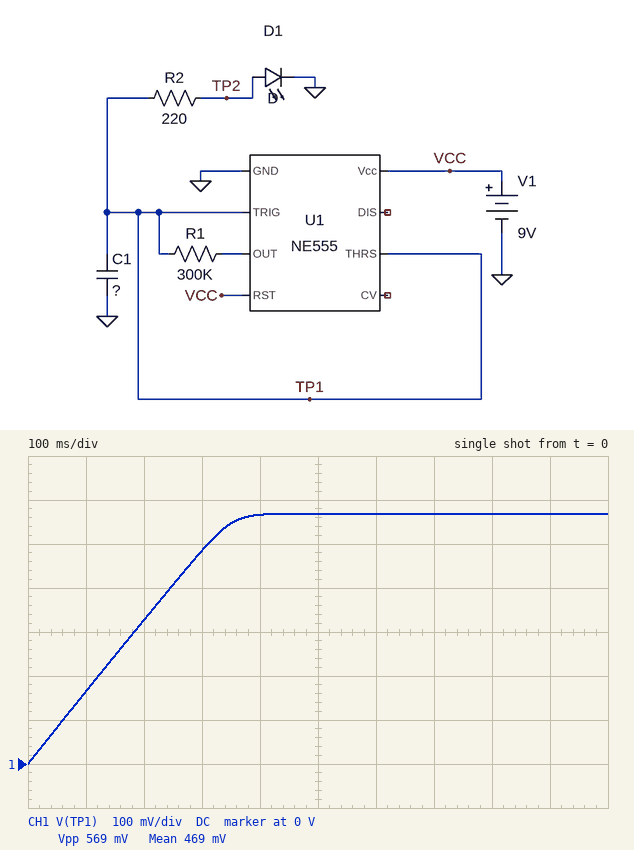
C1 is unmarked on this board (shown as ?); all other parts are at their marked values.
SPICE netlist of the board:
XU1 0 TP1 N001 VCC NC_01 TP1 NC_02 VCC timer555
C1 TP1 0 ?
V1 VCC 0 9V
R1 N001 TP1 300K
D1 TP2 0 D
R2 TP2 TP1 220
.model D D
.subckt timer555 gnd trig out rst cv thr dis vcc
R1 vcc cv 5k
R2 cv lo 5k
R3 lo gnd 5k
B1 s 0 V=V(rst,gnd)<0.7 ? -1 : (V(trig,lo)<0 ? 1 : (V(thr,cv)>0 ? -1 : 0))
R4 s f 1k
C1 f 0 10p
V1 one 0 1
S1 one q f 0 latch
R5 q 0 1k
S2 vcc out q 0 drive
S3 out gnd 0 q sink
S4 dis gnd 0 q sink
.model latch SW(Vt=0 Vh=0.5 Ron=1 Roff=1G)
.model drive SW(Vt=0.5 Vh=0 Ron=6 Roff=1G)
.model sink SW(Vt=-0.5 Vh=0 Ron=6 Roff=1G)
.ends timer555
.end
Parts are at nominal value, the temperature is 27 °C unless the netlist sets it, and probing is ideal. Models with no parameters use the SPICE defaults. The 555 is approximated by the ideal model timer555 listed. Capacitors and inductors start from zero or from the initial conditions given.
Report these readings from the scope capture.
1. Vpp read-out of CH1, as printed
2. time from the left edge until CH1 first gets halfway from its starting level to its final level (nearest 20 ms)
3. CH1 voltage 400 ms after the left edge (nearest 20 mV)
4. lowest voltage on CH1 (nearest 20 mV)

569 mV
180 ms
560 mV
0 V
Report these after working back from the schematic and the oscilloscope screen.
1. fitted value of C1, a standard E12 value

18 µF
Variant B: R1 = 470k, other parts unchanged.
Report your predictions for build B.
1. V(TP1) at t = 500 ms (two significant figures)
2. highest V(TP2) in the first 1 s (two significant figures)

510 mV
550 mV
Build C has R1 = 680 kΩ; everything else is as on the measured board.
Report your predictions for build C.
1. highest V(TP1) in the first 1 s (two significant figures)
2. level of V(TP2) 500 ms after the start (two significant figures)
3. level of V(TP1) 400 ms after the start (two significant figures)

540 mV
360 mV
290 mV
